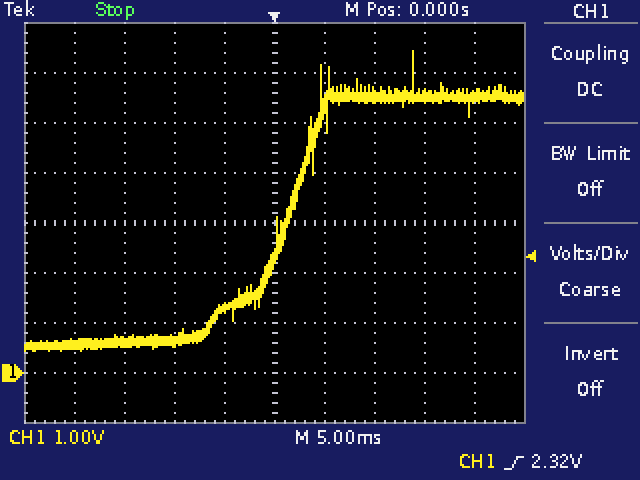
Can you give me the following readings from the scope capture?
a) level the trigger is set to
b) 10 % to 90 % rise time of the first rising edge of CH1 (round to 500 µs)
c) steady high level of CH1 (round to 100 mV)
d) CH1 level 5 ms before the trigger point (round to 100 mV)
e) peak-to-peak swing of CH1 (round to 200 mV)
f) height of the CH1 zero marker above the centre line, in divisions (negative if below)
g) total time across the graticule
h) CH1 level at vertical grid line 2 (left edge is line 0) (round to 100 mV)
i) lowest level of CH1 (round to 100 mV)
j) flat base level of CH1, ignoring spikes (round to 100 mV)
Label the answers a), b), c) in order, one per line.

a) 2.32 V
b) 10.5 ms
c) 5.5 V
d) 1.3 V
e) 6.0 V
f) -3.0 div
g) 50 ms
h) 600 mV
i) 400 mV
j) 600 mV
